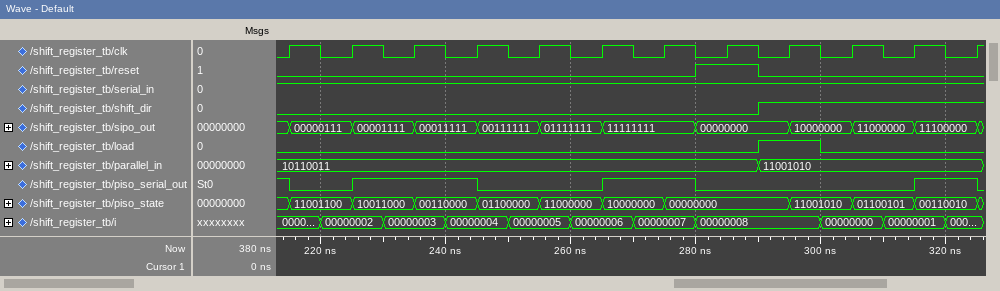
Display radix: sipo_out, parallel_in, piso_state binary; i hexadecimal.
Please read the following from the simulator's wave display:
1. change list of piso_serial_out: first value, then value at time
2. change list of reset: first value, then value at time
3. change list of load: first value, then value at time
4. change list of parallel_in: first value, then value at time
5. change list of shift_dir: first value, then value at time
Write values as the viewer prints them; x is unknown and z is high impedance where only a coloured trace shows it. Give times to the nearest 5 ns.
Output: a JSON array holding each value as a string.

["1, 0 at 215 ns, 1 at 225 ns, 0 at 245 ns, 1 at 265 ns, 0 at 280 ns, 1 at 315 ns, 0 at 325 ns", "0, 1 at 280 ns, 0 at 290 ns", "0, 1 at 290 ns, 0 at 300 ns", "10110011, 11001010 at 290 ns", "0, 1 at 290 ns"]
